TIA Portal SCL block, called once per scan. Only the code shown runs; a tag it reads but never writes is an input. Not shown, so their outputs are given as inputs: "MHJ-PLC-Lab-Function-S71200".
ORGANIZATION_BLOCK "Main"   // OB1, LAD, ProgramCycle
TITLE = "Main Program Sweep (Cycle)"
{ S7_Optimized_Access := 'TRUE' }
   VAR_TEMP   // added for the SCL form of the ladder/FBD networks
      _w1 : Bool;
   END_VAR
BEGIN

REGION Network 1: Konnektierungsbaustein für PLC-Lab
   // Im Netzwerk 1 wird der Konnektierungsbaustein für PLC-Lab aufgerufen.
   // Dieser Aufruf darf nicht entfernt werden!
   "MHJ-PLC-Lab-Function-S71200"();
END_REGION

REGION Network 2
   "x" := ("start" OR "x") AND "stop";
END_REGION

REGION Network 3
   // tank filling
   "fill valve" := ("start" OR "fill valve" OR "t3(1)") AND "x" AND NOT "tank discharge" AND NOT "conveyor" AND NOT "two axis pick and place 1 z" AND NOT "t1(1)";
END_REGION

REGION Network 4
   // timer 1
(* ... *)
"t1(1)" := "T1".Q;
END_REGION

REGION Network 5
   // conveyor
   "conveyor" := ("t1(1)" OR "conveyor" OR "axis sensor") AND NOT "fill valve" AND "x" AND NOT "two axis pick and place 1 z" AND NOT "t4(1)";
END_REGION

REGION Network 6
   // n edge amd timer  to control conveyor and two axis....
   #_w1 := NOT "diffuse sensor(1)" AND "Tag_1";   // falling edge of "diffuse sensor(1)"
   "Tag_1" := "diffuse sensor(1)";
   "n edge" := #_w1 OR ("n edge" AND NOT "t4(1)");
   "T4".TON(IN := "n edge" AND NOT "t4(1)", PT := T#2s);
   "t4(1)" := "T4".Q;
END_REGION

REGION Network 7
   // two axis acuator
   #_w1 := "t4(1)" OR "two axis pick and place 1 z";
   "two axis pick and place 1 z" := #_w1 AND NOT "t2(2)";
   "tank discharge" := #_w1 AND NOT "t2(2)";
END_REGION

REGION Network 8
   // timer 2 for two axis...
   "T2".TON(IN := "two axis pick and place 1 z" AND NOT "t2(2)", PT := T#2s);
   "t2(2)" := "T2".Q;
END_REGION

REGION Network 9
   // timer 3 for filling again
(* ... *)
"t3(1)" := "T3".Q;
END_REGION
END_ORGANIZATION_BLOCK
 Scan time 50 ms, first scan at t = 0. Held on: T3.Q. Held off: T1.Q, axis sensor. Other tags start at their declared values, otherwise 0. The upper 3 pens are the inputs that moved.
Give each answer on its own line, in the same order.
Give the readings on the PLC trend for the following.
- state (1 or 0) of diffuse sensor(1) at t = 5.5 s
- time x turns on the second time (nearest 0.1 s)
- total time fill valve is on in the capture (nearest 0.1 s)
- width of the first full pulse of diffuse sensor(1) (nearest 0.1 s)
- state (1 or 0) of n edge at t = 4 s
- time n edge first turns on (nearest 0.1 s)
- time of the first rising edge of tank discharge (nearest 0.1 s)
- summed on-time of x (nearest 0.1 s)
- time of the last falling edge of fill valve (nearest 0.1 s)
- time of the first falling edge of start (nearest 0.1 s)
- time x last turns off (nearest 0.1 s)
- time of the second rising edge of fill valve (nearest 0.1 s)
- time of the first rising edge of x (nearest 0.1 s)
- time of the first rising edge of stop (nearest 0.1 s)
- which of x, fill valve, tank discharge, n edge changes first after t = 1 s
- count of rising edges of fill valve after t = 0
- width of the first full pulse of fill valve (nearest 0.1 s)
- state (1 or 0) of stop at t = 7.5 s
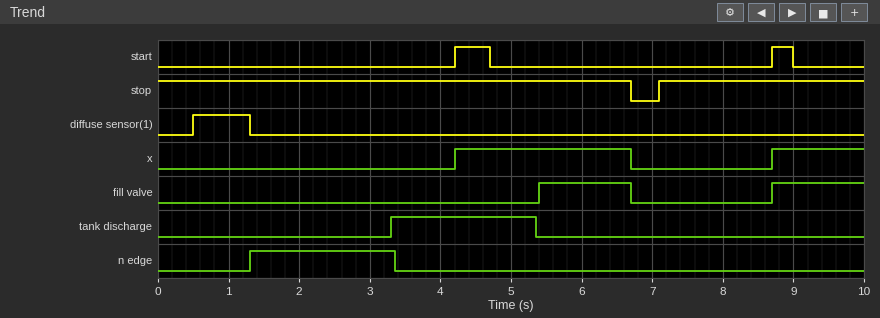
0
8.7 s
2.6 s
0.8 s
0
1.3 s
3.3 s
3.8 s
6.7 s
4.7 s
6.7 s
8.7 s
4.2 s
7.1 s
n edge
2
1.3 s
1
